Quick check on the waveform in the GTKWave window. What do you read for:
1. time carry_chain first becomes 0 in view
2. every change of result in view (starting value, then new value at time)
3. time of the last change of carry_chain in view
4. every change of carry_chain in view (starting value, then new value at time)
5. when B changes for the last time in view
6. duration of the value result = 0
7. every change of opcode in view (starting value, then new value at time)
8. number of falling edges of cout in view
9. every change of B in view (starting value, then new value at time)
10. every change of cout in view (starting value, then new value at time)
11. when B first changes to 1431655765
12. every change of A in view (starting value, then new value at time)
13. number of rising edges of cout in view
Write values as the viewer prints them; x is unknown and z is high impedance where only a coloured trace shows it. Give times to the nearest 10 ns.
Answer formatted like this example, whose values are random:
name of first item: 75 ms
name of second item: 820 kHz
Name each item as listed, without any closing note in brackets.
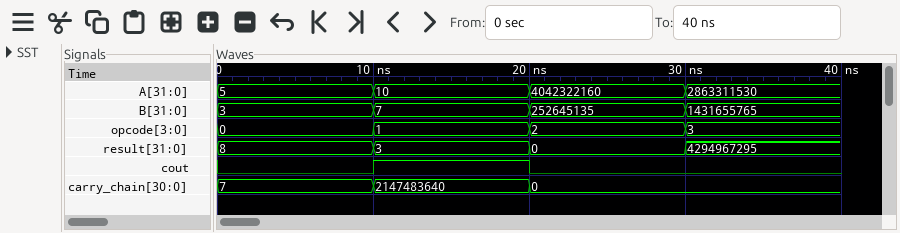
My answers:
time carry_chain first becomes 0 in view: 20 ns
every change of result in view: 8, 3 at 10 ns, 0 at 20 ns, 4294967295 at 30 ns
time of the last change of carry_chain in view: 20 ns
every change of carry_chain in view: 7, 2147483640 at 10 ns, 0 at 20 ns
when B changes for the last time in view: 30 ns
duration of the value result = 0: 10 ns
every change of opcode in view: 0, 1 at 10 ns, 2 at 20 ns, 3 at 30 ns
number of falling edges of cout in view: 1
every change of B in view: 3, 7 at 10 ns, 252645135 at 20 ns, 1431655765 at 30 ns
every change of cout in view: 0, 1 at 10 ns, 0 at 20 ns
when B first changes to 1431655765: 30 ns
every change of A in view: 5, 10 at 10 ns, 4042322160 at 20 ns, 2863311530 at 30 ns
number of rising edges of cout in view: 1
